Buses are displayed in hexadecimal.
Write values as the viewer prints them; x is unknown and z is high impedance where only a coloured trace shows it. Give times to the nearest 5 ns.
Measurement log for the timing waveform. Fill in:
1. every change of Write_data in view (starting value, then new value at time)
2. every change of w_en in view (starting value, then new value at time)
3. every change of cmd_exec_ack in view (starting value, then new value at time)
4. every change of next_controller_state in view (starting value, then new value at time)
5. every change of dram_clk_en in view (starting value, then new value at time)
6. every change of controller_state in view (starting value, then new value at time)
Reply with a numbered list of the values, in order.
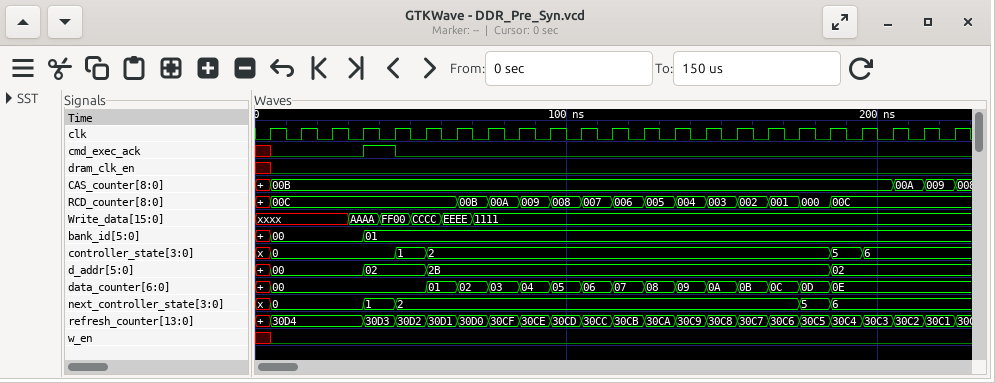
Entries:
1. xxxx, AAAA at 30 ns, FF00 at 40 ns, CCCC at 50 ns, EEEE at 60 ns, 1111 at 70 ns
2. x, 0 at 5 ns
3. x, 0 at 5 ns, 1 at 35 ns, 0 at 45 ns
4. x, 0 at 5 ns, 1 at 35 ns, 2 at 45 ns, 5 at 175 ns, 6 at 185 ns
5. x, 0 at 5 ns
6. x, 0 at 5 ns, 1 at 45 ns, 2 at 55 ns, 5 at 185 ns, 6 at 195 ns
